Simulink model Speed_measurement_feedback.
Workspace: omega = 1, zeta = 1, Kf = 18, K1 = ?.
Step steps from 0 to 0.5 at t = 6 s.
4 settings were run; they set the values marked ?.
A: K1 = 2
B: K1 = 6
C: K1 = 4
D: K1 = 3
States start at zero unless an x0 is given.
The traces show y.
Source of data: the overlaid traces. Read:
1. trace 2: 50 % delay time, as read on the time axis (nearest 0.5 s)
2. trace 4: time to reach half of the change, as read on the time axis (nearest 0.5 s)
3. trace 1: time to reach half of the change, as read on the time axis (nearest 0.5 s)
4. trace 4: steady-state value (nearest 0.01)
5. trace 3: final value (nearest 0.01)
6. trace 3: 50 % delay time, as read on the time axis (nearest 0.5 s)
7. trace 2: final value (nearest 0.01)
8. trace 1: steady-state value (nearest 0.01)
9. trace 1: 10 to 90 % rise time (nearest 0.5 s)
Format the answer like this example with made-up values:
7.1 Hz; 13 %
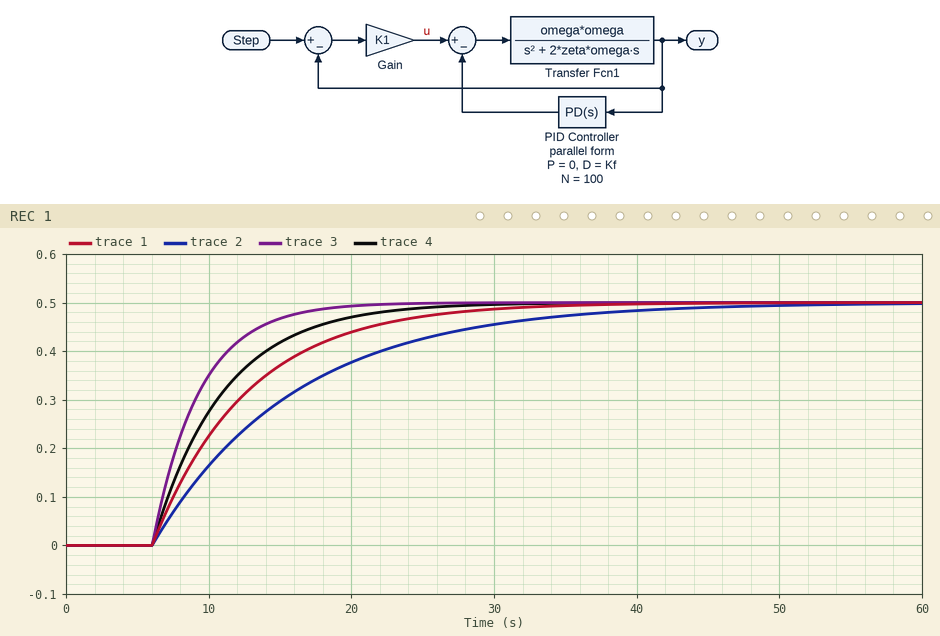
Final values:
13.0 s; 9.5 s; 10.5 s; 0.50; 0.50; 8.5 s; 0.50; 0.50; 14.5 s
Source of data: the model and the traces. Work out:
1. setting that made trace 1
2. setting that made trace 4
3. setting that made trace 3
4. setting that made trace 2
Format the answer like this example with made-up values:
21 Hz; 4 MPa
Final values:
D; C; B; A
